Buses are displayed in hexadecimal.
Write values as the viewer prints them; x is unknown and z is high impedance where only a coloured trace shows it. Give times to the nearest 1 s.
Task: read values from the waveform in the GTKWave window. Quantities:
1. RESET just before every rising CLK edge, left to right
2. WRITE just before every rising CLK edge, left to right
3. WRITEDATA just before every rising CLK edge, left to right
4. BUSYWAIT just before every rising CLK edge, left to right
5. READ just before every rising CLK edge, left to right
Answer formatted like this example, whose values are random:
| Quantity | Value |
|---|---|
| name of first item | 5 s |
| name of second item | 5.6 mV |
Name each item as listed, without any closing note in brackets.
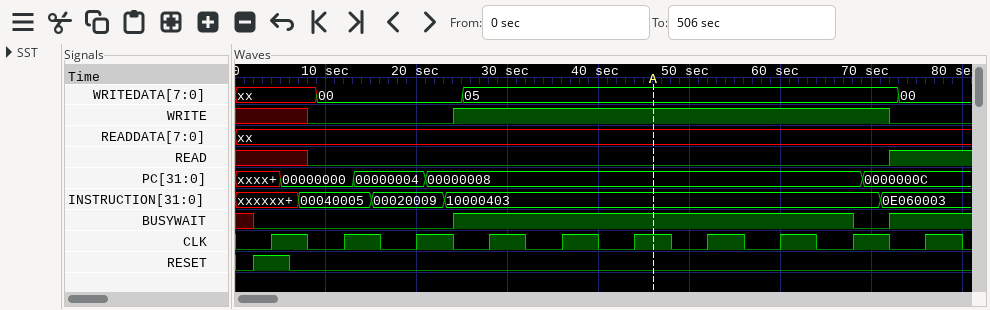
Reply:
| Quantity | Value |
|---|---|
| RESET just before every rising CLK edge, left to right | 1 0 0 0 0 0 0 0 0 0 |
| WRITE just before every rising CLK edge, left to right | x 0 0 1 1 1 1 1 1 0 |
| WRITEDATA just before every rising CLK edge, left to right | xx, 00, 00, 05, 05, 05, 05, 05, 05, 00 |
| BUSYWAIT just before every rising CLK edge, left to right | 0 0 0 1 1 1 1 1 1 1 |
| READ just before every rising CLK edge, left to right | x 0 0 0 0 0 0 0 0 1 |
